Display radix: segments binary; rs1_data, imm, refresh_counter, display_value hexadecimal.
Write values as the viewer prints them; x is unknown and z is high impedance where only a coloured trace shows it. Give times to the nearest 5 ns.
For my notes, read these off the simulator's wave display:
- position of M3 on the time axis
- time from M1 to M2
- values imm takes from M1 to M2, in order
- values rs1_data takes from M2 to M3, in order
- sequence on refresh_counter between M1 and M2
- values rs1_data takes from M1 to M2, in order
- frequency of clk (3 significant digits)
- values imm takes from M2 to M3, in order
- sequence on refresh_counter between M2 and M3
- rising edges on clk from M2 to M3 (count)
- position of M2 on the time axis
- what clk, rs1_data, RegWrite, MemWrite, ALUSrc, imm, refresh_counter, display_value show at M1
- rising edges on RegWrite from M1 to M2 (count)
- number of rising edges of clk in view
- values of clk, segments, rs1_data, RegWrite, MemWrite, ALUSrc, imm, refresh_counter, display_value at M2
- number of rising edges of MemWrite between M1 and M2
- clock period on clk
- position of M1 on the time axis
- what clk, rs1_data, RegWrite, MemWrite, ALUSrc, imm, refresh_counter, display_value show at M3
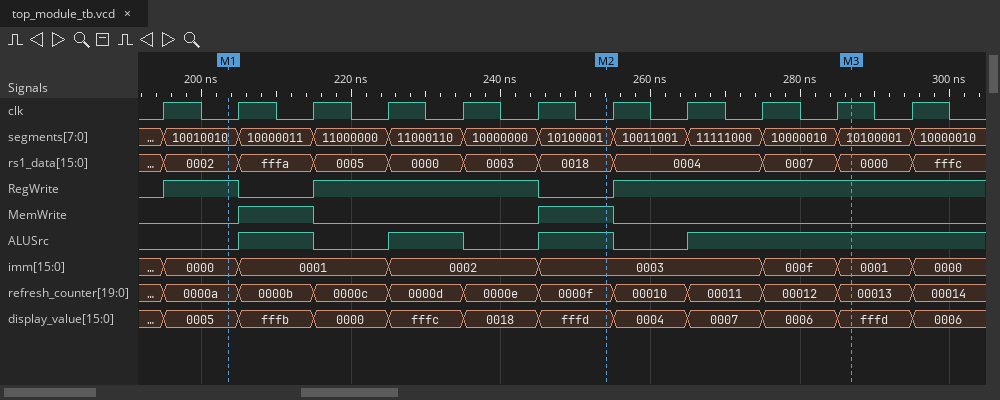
285 ns
50 ns
0000, 0001, 0002, 0003
0018, 0004, 0007, 0000
0000a, 0000b, 0000c, 0000d, 0000e, 0000f
0002, fffa, 0005, 0000, 0003, 0018
100 MHz
0003, 000f, 0001
0000f, 00010, 00011, 00012, 00013
4
255 ns
clk=0, rs1_data=0002, RegWrite=1, MemWrite=0, ALUSrc=0, imm=0000, refresh_counter=0000a, display_value=0005
1
11
clk=0, segments=10100001, rs1_data=0018, RegWrite=0, MemWrite=1, ALUSrc=1, imm=0003, refresh_counter=0000f, display_value=fffd
2
10 ns
205 ns
clk=1, rs1_data=0000, RegWrite=1, MemWrite=0, ALUSrc=1, imm=0001, refresh_counter=00013, display_value=fffd
